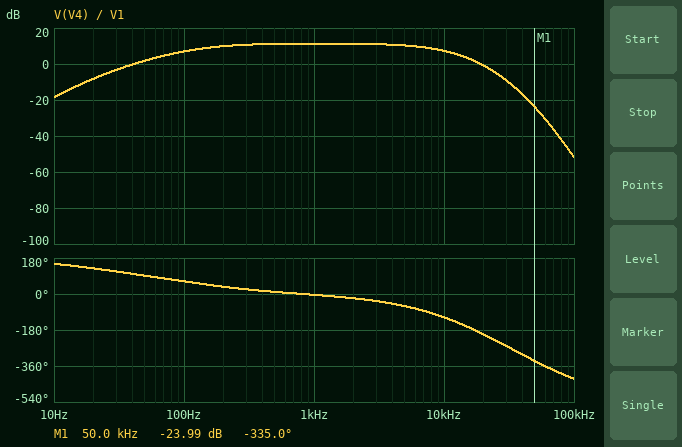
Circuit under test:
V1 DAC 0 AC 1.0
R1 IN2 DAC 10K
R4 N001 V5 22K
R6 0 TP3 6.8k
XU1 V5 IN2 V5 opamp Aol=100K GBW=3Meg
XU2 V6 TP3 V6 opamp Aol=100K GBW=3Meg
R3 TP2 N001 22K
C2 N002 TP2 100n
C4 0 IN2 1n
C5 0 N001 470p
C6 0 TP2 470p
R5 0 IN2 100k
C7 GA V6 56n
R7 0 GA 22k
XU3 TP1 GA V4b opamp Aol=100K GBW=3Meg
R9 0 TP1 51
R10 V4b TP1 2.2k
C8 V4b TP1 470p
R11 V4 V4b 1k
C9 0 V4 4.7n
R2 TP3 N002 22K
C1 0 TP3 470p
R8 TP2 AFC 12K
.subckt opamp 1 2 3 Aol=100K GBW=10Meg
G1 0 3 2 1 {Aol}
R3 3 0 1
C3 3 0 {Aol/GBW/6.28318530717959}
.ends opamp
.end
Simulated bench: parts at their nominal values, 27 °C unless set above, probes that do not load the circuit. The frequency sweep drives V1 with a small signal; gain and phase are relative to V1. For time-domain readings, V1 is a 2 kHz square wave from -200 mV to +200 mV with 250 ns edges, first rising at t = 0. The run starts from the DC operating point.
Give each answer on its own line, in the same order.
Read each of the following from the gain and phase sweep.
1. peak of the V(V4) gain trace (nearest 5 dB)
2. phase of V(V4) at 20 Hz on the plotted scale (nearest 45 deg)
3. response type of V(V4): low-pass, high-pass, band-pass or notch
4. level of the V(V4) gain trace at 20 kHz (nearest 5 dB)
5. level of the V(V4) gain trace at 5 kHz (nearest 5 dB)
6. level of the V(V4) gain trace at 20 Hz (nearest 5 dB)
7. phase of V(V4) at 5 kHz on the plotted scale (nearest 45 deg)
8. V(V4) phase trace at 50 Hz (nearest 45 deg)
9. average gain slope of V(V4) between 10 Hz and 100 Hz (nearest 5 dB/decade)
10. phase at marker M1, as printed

10 dB
135 deg
band-pass
0 dB
10 dB
-10 dB
-45 deg
90 deg
25 dB/decade
-335.0 deg
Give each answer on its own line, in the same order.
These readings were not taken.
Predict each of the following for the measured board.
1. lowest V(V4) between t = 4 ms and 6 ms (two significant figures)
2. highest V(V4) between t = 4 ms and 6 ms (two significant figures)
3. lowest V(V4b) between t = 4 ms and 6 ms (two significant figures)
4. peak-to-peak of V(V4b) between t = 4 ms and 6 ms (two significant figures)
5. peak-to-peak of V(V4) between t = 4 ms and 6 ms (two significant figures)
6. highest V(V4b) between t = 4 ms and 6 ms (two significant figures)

-840 mV
730 mV
-840 mV
1.6 V
1.6 V
730 mV
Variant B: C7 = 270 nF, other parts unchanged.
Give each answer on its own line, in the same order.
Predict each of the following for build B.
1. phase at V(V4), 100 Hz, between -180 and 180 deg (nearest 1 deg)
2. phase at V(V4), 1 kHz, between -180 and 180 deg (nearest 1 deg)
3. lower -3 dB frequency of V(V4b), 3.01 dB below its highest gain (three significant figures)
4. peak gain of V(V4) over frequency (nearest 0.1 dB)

26 deg
-10 deg
37.6 Hz
11.4 dB
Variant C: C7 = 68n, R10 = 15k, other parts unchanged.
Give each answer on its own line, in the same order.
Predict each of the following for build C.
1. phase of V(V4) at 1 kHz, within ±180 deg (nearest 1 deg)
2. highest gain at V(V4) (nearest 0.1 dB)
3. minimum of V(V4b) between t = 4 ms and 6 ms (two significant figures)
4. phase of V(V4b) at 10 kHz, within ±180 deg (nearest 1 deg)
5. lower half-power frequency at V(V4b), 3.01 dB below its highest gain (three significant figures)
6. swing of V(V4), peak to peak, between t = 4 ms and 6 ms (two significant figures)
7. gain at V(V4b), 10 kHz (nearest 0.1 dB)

-12 deg
27.8 dB
-5.5 V
-143 deg
107 Hz
10 V
19.6 dB
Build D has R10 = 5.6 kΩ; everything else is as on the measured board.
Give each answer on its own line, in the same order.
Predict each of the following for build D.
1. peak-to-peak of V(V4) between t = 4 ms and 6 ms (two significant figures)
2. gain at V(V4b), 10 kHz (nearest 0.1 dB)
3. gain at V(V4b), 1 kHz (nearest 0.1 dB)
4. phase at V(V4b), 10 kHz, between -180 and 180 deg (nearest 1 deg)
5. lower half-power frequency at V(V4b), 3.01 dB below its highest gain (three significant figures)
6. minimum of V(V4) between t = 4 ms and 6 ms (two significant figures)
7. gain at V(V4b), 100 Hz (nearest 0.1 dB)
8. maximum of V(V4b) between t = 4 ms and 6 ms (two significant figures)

3.9 V
14.8 dB
19.3 dB
-116 deg
129 Hz
-2.1 V
15.0 dB
1.8 V
